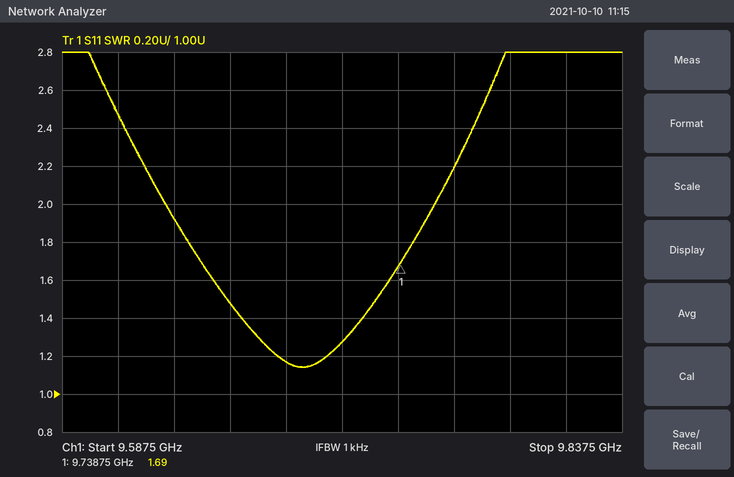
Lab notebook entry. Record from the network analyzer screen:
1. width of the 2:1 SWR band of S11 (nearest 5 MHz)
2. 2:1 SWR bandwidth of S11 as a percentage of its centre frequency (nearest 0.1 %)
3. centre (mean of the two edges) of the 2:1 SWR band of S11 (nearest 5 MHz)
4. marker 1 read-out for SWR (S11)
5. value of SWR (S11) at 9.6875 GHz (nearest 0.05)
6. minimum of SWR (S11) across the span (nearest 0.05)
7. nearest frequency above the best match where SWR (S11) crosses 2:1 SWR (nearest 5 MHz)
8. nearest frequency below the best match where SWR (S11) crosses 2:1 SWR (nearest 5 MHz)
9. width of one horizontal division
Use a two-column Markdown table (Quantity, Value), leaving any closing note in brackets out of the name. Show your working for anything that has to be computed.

| Quantity | Value |
|---|---|
| width of the 2:1 SWR band of S11 | 9.755 GHz − 9.635 GHz = 120 MHz |
| 2:1 SWR bandwidth of S11 as a percentage of its centre frequency | 120 MHz / 9.695 GHz ≈ 1.2 % |
| centre (mean of the two edges) of the 2:1 SWR band of S11 | 9.695 GHz |
| marker 1 read-out for SWR | 1.69 |
| value of SWR (S11) at 9.6875 GHz | 1.15 |
| minimum of SWR (S11) across the span | 1.15 |
| nearest frequency above the best match where SWR (S11) crosses 2:1 SWR | 9.755 GHz |
| nearest frequency below the best match where SWR (S11) crosses 2:1 SWR | 9.635 GHz |
| width of one horizontal division | 25 MHz |
